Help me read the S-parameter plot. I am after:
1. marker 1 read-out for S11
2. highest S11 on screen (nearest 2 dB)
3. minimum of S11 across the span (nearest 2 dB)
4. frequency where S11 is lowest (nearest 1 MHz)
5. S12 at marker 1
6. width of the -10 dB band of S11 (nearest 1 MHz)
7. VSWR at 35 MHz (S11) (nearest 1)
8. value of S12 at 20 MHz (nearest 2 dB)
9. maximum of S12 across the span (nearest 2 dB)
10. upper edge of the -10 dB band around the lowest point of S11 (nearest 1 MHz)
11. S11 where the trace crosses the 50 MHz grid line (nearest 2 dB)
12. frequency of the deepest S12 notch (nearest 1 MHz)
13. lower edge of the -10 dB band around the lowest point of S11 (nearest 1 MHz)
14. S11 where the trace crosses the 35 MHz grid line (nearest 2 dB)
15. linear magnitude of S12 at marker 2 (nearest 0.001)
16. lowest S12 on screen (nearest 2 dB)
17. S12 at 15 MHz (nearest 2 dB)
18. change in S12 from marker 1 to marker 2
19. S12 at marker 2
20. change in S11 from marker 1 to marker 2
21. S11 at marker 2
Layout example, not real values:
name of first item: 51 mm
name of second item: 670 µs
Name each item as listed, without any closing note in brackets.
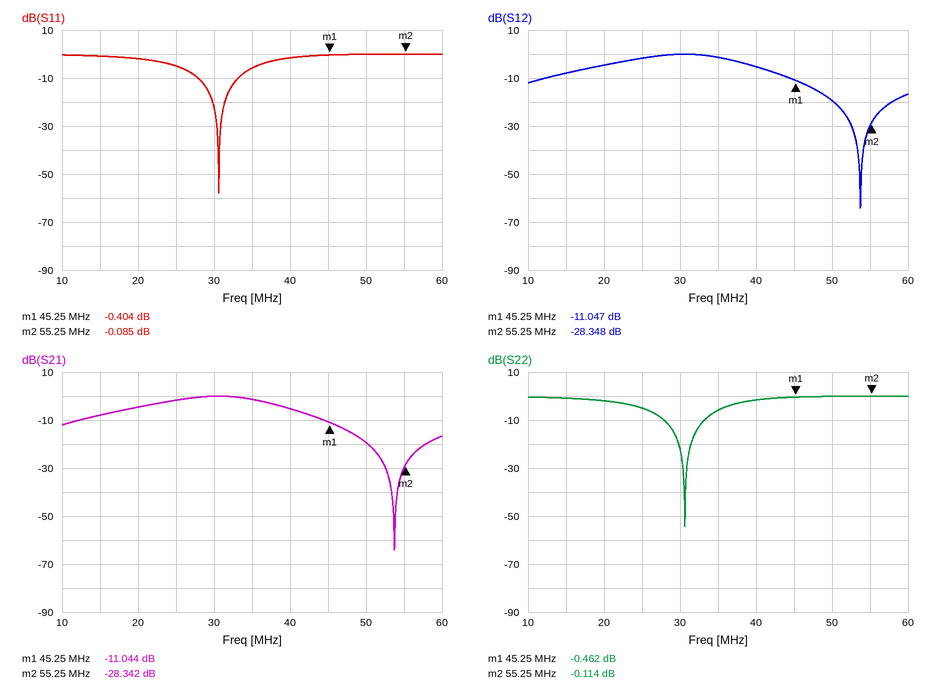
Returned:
marker 1 read-out for S11: -0.404 dB
highest S11 on screen: 0 dB
minimum of S11 across the span: -58 dB
frequency where S11 is lowest: 31 MHz
S12 at marker 1: -11.047 dB
width of the -10 dB band of S11: 5 MHz
VSWR at 35 MHz (S11): 3
value of S12 at 20 MHz: -4 dB
maximum of S12 across the span: 0 dB
upper edge of the -10 dB band around the lowest point of S11: 33 MHz
S11 where the trace crosses the 50 MHz grid line: 0 dB
frequency of the deepest S12 notch: 54 MHz
lower edge of the -10 dB band around the lowest point of S11: 28 MHz
S11 where the trace crosses the 35 MHz grid line: -6 dB
linear magnitude of S12 at marker 2: 0.038
lowest S12 on screen: -64 dB
S12 at 15 MHz: -8 dB
change in S12 from marker 1 to marker 2: -17.301 dB
S12 at marker 2: -28.348 dB
change in S11 from marker 1 to marker 2: 0.319 dB
S11 at marker 2: -0.085 dB
